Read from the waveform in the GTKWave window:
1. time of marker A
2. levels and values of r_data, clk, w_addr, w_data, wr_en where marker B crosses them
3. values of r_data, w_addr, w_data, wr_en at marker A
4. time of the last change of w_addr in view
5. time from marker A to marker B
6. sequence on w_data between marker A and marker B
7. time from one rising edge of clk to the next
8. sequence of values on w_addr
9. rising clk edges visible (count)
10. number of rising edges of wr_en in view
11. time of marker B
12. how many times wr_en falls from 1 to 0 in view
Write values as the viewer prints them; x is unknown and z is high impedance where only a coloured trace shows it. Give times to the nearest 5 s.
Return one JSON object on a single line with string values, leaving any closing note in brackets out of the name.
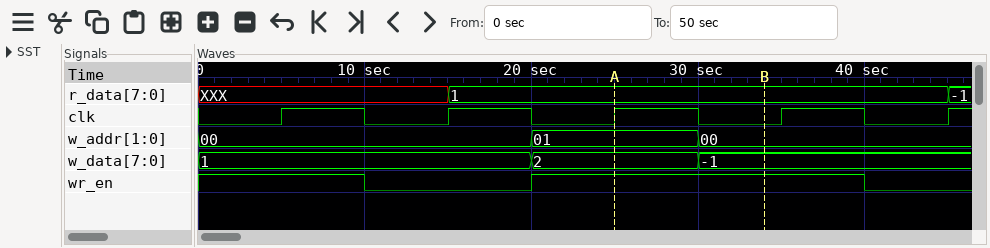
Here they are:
{"time of marker A": "25 s", "levels and values of r_data, clk, w_addr, w_data, wr_en where marker B crosses them": "r_data=1, clk=0, w_addr=00, w_data=-1, wr_en=1", "values of r_data, w_addr, w_data, wr_en at marker A": "r_data=1, w_addr=01, w_data=2, wr_en=1", "time of the last change of w_addr in view": "30 s", "time from marker A to marker B": "10 s", "sequence on w_data between marker A and marker B": "2, -1", "time from one rising edge of clk to the next": "10 s", "sequence of values on w_addr": "00, 01, 00", "rising clk edges visible": "5", "number of rising edges of wr_en in view": "1", "time of marker B": "35 s", "how many times wr_en falls from 1 to 0 in view": "2"}
